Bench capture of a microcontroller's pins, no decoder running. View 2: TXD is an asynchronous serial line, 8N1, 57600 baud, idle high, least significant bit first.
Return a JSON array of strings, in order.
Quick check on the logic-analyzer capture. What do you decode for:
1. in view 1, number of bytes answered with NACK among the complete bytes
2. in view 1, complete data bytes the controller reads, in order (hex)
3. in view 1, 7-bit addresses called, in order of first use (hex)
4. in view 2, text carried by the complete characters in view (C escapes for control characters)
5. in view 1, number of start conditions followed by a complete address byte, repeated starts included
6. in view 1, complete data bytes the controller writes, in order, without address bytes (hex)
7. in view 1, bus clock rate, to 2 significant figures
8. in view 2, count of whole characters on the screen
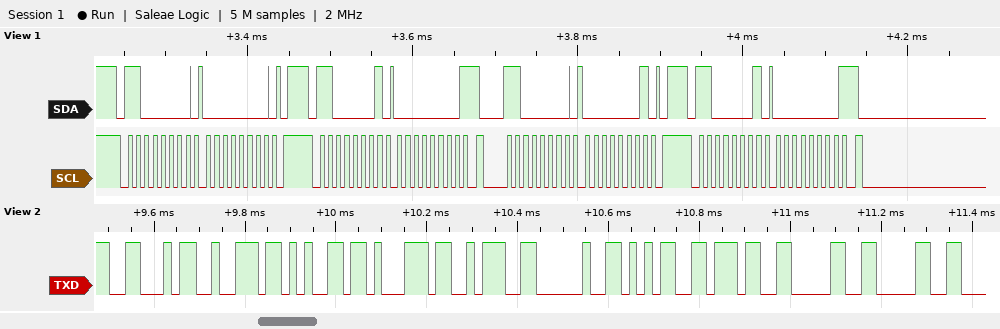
["2", "00 00", "0x60", "\"Freq: 5700\"", "4", "00 01", "100 kHz", "10"]
